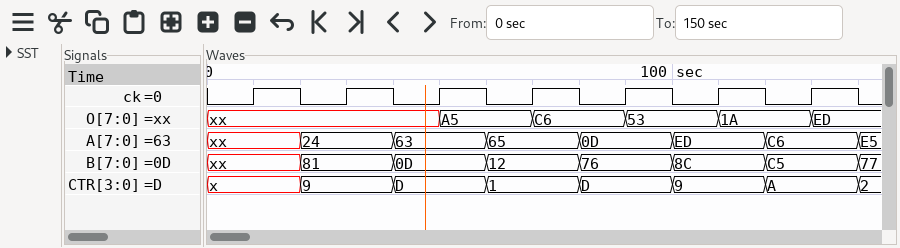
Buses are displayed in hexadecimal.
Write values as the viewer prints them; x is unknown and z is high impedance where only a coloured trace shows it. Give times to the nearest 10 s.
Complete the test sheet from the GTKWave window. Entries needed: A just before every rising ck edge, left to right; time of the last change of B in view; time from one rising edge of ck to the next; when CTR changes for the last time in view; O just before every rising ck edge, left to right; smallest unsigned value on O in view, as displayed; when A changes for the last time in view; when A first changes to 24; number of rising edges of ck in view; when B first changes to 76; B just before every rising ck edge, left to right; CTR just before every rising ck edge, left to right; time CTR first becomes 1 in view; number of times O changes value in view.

xx, 24, 63, 65, 0D, ED, C6
140 s
20 s
140 s
xx, xx, xx, A5, C6, 53, 1A
1A
140 s
20 s
7
80 s
xx, 81, 0D, 12, 76, 8C, C5
x, 9, D, 1, D, 9, A
60 s
5
